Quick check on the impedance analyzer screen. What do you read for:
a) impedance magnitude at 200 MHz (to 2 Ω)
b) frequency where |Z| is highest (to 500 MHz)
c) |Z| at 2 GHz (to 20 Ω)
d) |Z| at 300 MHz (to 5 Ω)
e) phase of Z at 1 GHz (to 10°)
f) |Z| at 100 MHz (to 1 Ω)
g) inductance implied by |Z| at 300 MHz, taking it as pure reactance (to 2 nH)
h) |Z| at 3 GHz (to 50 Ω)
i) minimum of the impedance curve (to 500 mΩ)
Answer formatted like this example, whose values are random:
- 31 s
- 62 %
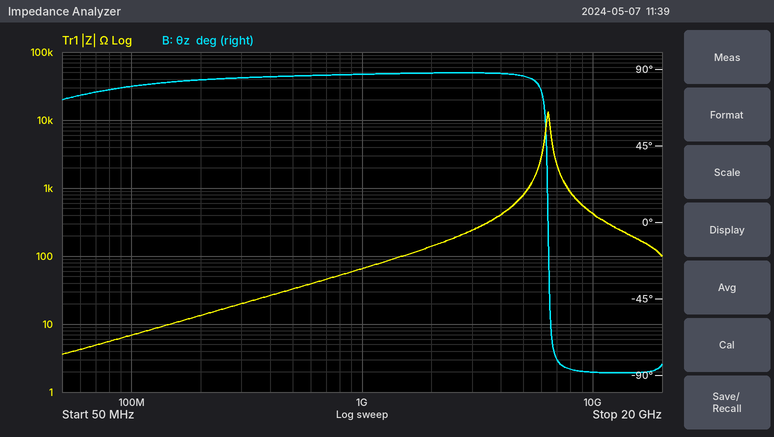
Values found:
- 14 Ω
- 6.5 GHz
- 140 Ω
- 20 Ω
- 90°
- 7 Ω
- 10 nH
- 250 Ω
- 3.5 Ω
